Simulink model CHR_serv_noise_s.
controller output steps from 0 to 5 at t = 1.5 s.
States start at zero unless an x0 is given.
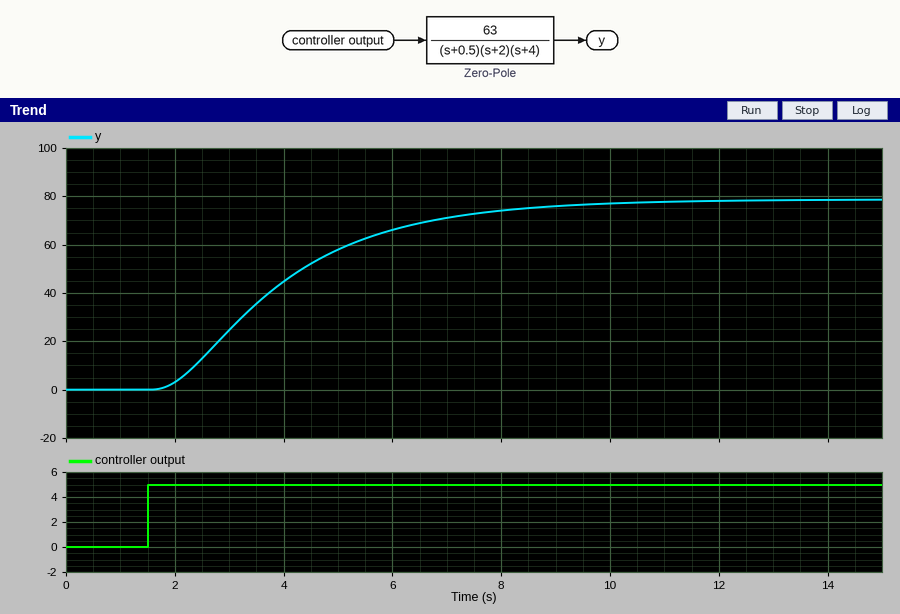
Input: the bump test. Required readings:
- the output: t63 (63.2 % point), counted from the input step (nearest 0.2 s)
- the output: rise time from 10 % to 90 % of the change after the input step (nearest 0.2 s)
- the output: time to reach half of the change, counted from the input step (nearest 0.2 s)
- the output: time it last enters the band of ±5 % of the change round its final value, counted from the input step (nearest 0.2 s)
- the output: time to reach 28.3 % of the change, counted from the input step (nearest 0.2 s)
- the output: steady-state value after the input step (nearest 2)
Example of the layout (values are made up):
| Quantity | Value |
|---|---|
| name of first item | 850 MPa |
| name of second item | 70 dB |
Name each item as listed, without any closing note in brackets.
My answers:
| Quantity | Value |
|---|---|
| the output: t63 (63.2 % point), counted from the input step | 2.8 s |
| the output: rise time from 10 % to 90 % of the change after the input step | 4.6 s |
| the output: time to reach half of the change, counted from the input step | 2.2 s |
| the output: time it last enters the band of ±5 % of the change round its final value, counted from the input step | 6.8 s |
| the output: time to reach 28.3 % of the change, counted from the input step | 1.4 s |
| the output: steady-state value after the input step | 78 |
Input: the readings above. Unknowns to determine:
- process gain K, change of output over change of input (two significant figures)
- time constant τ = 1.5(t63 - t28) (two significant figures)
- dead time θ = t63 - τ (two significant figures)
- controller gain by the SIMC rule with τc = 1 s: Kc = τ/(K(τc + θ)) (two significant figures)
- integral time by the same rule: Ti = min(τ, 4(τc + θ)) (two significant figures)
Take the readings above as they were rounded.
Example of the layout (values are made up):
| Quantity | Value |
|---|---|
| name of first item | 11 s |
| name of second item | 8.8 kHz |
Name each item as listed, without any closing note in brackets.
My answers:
| Quantity | Value |
|---|---|
| process gain K, change of output over change of input | 16 |
| time constant τ = 1.5(t63 - t28) | 2.1 s |
| dead time θ = t63 - τ | 0.70 s |
| controller gain by the SIMC rule with τc = 1 s: Kc = τ/(K(τc + θ)) | 0.077 |
| integral time by the same rule: Ti = min(τ, 4(τc + θ)) | 2.1 s |
